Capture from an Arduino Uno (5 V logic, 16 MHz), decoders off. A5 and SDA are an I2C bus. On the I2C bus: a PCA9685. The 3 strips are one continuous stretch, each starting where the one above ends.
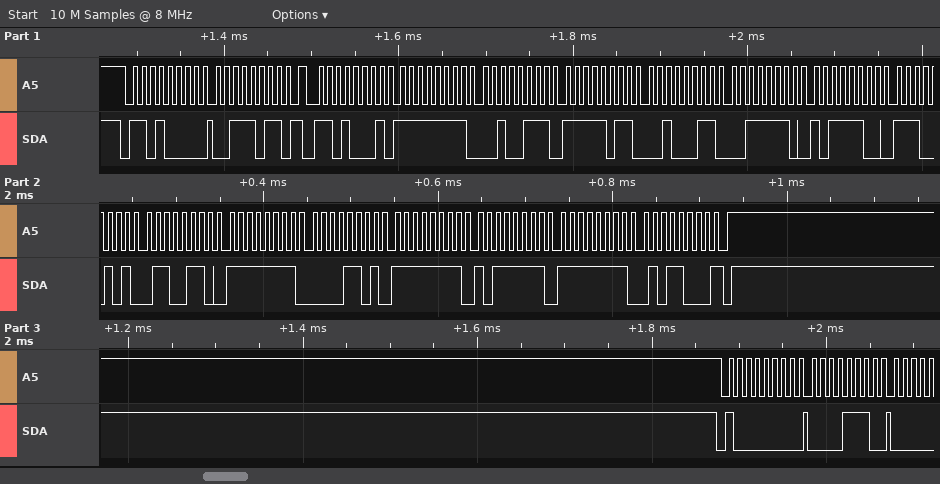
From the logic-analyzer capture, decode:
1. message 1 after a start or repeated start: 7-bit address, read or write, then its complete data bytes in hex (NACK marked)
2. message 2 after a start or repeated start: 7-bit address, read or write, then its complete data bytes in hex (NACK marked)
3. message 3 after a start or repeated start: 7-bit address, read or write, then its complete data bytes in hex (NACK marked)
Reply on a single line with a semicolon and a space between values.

0x68 write: 3B; 0x68 read: FF 27 FB 23 3E BC E5 66 FF 0D FF BF FF 58 NACK; 0x40 write: 0E
